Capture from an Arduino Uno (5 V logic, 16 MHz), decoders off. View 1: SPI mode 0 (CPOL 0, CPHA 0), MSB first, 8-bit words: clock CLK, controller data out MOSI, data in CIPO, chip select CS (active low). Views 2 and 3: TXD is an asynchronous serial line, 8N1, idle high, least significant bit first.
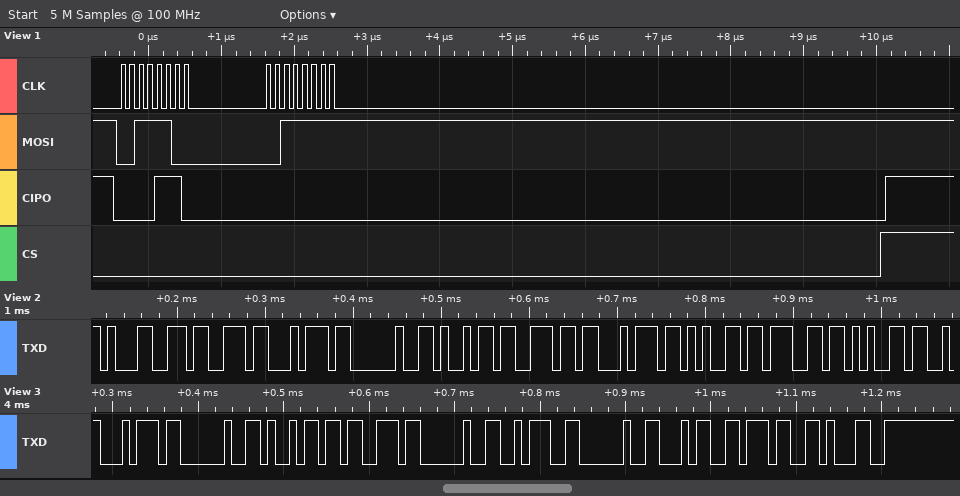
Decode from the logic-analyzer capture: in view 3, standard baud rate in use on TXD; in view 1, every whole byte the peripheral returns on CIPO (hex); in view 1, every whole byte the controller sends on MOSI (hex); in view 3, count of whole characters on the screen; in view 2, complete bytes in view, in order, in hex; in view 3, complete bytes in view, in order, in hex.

115200 baud
0x0E 0x00
0x3C 0x3F
10
31 73 74 20 69 6E 74 65 67 65
74 20 69 73 20 3A 20 34 37 31
